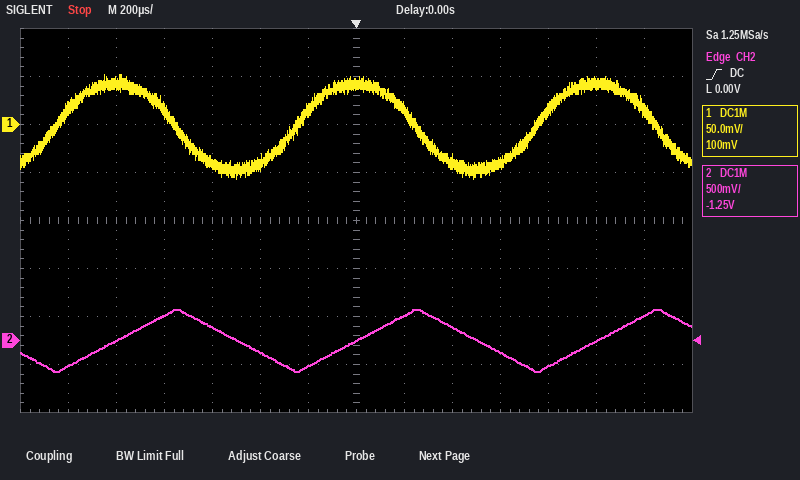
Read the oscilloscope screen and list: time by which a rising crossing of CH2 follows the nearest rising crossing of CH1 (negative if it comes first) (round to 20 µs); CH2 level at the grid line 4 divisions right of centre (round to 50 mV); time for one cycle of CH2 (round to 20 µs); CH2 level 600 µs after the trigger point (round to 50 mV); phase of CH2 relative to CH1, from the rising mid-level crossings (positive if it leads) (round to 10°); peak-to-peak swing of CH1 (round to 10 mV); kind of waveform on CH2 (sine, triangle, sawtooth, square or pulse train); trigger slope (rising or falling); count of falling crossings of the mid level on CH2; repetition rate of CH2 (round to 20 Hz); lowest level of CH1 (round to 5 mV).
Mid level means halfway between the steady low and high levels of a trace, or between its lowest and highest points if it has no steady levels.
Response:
+260 µs
-250 mV
1.00 ms
-100 mV
-90°
110 mV
triangle
rising
2
1.00 kHz
-55 mV
